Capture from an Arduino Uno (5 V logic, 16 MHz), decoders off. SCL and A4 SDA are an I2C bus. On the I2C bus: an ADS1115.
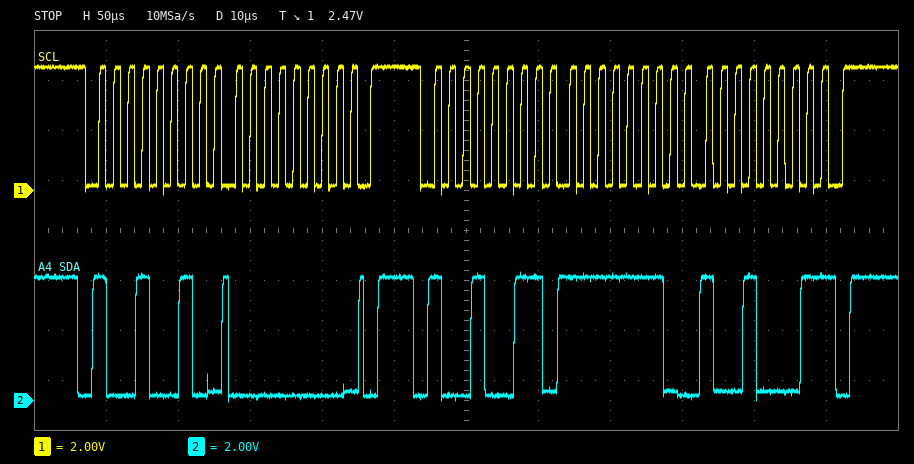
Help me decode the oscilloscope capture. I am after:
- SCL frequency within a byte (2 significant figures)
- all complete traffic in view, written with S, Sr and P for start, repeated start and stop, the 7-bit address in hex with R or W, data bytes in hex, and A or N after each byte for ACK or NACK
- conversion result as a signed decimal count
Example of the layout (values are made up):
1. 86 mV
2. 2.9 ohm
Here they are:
1. 100 kHz
2. S 49W A 00 A P S 49R A FE A 91 N P
3. -367
